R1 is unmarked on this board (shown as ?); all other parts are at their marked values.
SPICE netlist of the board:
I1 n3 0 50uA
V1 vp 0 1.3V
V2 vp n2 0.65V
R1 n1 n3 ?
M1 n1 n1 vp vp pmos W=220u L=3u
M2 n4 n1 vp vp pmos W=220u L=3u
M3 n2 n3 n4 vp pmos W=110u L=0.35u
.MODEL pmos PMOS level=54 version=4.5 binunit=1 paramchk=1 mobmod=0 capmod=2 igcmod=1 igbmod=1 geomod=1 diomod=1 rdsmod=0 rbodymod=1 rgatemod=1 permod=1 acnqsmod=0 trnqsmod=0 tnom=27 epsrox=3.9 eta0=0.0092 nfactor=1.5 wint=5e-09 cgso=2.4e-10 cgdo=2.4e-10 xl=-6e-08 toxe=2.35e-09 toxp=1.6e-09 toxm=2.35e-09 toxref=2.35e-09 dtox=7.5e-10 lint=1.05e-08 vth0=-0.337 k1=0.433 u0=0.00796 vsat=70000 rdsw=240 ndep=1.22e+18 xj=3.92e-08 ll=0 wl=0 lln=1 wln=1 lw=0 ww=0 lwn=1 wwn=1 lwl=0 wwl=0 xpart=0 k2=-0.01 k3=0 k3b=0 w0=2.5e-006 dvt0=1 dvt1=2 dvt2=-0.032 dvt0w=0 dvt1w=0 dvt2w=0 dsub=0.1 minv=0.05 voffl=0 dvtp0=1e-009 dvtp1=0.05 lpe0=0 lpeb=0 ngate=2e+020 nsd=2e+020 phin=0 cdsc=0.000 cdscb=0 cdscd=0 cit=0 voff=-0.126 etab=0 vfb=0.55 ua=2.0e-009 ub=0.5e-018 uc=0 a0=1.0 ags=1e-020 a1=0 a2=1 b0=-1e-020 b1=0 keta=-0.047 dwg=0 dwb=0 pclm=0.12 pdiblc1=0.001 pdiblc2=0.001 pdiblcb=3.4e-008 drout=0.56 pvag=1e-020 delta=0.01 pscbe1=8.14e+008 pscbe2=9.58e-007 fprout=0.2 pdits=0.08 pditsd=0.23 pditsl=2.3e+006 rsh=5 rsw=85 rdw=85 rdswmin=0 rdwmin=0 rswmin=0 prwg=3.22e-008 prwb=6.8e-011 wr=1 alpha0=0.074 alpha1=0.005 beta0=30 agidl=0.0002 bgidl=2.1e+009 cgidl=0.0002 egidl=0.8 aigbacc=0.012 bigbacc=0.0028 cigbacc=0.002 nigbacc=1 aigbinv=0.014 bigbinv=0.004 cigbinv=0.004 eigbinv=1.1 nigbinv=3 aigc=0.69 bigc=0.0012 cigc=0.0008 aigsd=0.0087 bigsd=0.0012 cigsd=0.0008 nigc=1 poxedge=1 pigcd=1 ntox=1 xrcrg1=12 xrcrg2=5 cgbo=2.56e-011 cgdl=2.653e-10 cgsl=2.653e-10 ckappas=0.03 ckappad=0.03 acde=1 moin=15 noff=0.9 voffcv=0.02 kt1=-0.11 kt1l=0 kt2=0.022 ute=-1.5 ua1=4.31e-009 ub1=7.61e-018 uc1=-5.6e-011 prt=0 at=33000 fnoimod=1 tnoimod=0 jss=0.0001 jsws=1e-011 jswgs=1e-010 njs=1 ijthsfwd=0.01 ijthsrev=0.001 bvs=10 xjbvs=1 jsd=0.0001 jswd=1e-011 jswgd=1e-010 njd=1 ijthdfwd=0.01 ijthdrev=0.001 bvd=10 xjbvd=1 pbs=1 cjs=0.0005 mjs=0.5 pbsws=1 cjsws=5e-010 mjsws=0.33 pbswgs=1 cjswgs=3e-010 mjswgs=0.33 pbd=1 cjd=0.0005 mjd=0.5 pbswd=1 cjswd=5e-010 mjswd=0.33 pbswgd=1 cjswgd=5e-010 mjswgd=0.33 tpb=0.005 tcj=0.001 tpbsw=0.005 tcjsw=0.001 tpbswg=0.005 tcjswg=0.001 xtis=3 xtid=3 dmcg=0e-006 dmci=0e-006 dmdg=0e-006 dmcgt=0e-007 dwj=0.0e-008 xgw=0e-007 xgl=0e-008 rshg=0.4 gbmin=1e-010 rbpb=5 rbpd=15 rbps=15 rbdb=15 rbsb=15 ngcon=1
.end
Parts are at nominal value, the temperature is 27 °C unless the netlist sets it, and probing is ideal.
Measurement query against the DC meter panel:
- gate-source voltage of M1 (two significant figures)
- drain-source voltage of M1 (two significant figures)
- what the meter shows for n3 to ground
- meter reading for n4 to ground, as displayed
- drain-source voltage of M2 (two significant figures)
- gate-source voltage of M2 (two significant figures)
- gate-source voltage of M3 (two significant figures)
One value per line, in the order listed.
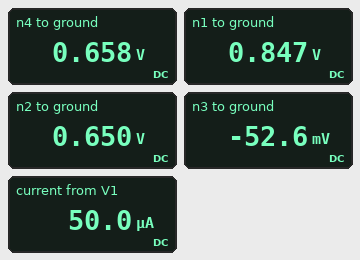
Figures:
-450 mV
-450 mV
-52.6 mV
0.658 V
-640 mV
-450 mV
-710 mV
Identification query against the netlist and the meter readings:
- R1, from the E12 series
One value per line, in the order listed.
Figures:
18 kΩ
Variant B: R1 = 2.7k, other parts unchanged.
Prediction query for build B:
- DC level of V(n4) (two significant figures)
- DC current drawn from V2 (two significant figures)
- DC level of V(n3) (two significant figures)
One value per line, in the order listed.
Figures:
1.1 V
49 µA
710 mV
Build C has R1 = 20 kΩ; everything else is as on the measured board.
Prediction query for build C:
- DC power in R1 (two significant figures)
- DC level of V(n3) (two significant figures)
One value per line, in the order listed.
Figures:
50 µW
-150 mV
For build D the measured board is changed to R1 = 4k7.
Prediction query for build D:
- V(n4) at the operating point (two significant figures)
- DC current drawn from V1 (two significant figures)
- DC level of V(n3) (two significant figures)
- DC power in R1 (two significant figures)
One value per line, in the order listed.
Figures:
1.0 V
50 µA
610 mV
12 µW
